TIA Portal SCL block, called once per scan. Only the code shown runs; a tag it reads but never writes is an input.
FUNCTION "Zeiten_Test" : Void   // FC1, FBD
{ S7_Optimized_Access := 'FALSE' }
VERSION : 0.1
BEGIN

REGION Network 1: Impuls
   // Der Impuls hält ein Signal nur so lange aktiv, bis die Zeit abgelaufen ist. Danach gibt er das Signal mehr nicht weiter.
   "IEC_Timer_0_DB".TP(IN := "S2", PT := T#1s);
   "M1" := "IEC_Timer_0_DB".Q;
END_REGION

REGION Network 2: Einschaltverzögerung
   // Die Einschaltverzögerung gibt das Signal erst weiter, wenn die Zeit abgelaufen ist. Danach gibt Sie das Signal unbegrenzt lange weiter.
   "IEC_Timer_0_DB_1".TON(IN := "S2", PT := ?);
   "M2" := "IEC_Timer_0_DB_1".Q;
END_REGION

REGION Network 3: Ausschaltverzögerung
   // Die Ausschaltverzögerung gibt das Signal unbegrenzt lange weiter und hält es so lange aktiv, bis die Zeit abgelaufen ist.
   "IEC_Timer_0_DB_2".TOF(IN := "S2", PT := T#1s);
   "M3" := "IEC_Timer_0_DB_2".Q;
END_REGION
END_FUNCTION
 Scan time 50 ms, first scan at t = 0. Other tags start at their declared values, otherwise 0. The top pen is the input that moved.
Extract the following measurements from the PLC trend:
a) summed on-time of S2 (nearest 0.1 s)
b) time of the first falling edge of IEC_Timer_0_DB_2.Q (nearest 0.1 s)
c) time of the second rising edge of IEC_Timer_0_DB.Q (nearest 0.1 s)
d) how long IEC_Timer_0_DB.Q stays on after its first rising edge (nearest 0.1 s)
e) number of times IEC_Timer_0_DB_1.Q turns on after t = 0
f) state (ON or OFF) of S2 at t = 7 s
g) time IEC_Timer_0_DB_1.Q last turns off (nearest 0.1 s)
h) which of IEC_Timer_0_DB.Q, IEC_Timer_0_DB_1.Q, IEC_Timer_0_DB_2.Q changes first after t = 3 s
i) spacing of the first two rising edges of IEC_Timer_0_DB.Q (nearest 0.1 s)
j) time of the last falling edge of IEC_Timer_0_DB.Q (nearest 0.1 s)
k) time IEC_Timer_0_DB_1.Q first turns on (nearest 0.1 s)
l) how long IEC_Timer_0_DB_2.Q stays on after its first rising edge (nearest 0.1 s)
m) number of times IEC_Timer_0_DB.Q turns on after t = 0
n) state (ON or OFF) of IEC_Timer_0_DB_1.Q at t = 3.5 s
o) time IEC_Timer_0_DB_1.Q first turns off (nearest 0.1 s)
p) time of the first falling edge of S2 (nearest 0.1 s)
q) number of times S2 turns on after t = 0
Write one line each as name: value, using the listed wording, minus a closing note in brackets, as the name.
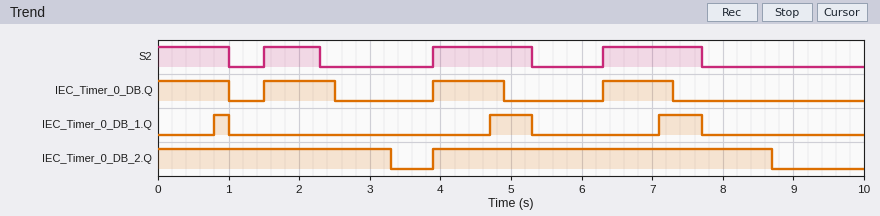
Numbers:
summed on-time of S2: 4.6 s
time of the first falling edge of IEC_Timer_0_DB_2.Q: 3.3 s
time of the second rising edge of IEC_Timer_0_DB.Q: 3.9 s
how long IEC_Timer_0_DB.Q stays on after its first rising edge: 1.0 s
number of times IEC_Timer_0_DB_1.Q turns on after t = 0: 3
state (ON or OFF) of S2 at t = 7 s: ON
time IEC_Timer_0_DB_1.Q last turns off: 7.7 s
which of IEC_Timer_0_DB.Q, IEC_Timer_0_DB_1.Q, IEC_Timer_0_DB_2.Q changes first after t = 3 s: IEC_Timer_0_DB_2.Q
spacing of the first two rising edges of IEC_Timer_0_DB.Q: 2.4 s
time of the last falling edge of IEC_Timer_0_DB.Q: 7.3 s
time IEC_Timer_0_DB_1.Q first turns on: 0.8 s
how long IEC_Timer_0_DB_2.Q stays on after its first rising edge: 4.8 s
number of times IEC_Timer_0_DB.Q turns on after t = 0: 3
state (ON or OFF) of IEC_Timer_0_DB_1.Q at t = 3.5 s: OFF
time IEC_Timer_0_DB_1.Q first turns off: 1.0 s
time of the first falling edge of S2: 1.0 s
number of times S2 turns on after t = 0: 3
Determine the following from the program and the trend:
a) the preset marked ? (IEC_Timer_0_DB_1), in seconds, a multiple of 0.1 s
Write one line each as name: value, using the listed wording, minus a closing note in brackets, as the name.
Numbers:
the preset marked ? (IEC_Timer_0_DB_1), in seconds, a multiple of 0.1 s: 0.8 s
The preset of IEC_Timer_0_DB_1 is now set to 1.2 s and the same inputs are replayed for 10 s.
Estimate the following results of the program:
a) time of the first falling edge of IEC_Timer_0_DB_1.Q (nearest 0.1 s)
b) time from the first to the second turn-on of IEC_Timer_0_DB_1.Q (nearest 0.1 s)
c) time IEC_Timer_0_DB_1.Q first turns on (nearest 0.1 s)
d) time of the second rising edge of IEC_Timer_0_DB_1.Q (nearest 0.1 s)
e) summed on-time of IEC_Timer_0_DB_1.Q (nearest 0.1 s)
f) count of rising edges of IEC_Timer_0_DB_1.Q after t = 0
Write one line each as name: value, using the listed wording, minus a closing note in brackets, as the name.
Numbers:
time of the first falling edge of IEC_Timer_0_DB_1.Q: 5.3 s
time from the first to the second turn-on of IEC_Timer_0_DB_1.Q: 2.4 s
time IEC_Timer_0_DB_1.Q first turns on: 5.1 s
time of the second rising edge of IEC_Timer_0_DB_1.Q: 7.5 s
summed on-time of IEC_Timer_0_DB_1.Q: 0.4 s
count of rising edges of IEC_Timer_0_DB_1.Q after t = 0: 2
